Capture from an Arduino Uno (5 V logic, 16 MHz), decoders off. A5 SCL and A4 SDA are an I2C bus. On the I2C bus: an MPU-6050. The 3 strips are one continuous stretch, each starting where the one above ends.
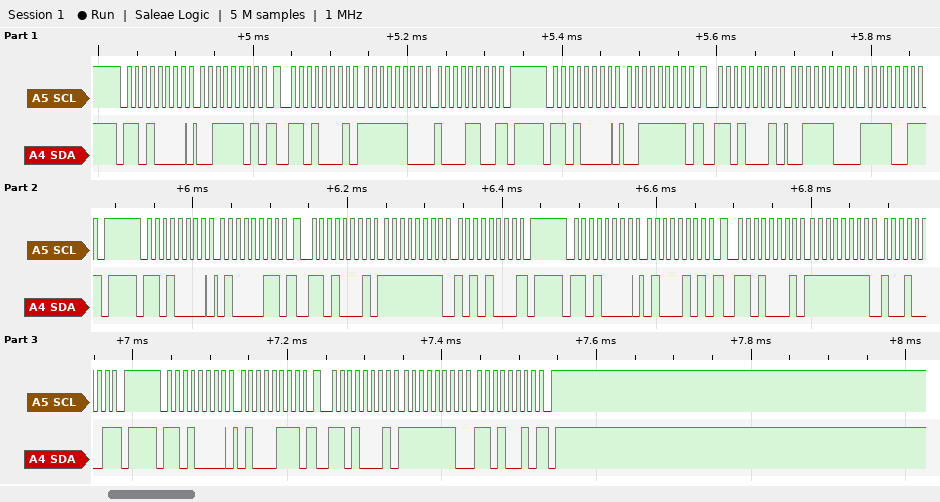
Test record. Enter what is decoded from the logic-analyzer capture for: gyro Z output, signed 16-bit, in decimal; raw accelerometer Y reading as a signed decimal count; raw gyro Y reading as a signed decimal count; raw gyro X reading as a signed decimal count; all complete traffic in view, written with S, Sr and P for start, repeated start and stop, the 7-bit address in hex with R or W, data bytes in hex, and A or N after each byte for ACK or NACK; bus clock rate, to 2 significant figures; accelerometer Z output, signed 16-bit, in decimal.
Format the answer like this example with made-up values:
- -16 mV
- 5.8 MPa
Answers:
- -302
- -884
- -111
- -88
- S 68W A 3D A Sr 68R A FC A 8C N P S 68W A 3F A Sr 68R A 3C A F3 N P S 68W A 43 A Sr 68R A FF A A8 N P S 68W A 45 A Sr 68R A FF A 91 N P S 68W A 47 A Sr 68R A FE A D2 N P
- 100 kHz
- 15603
